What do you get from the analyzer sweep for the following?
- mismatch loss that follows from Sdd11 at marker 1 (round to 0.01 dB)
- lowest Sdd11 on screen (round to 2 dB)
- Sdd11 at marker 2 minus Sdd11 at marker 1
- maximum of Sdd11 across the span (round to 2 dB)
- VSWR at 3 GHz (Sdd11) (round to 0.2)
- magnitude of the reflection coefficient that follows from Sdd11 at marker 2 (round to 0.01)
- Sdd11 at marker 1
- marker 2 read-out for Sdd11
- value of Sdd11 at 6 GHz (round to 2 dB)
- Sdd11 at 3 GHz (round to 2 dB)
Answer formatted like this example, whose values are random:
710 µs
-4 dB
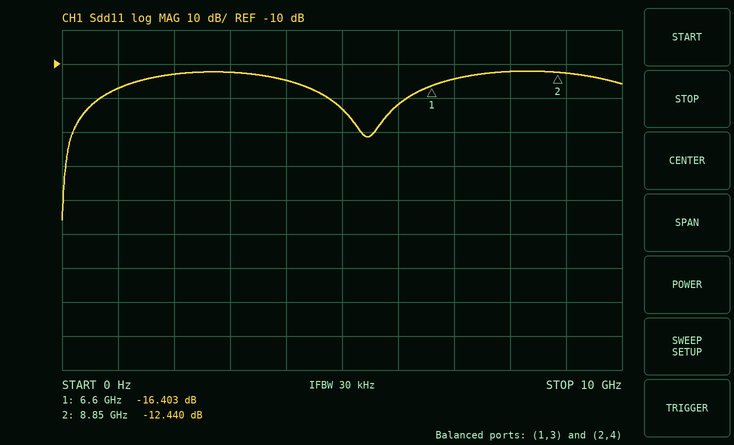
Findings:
0.10 dB
-56 dB
3.963 dB
-12 dB
1.6
0.24
-16.403 dB
-12.440 dB
-22 dB
-12 dB
